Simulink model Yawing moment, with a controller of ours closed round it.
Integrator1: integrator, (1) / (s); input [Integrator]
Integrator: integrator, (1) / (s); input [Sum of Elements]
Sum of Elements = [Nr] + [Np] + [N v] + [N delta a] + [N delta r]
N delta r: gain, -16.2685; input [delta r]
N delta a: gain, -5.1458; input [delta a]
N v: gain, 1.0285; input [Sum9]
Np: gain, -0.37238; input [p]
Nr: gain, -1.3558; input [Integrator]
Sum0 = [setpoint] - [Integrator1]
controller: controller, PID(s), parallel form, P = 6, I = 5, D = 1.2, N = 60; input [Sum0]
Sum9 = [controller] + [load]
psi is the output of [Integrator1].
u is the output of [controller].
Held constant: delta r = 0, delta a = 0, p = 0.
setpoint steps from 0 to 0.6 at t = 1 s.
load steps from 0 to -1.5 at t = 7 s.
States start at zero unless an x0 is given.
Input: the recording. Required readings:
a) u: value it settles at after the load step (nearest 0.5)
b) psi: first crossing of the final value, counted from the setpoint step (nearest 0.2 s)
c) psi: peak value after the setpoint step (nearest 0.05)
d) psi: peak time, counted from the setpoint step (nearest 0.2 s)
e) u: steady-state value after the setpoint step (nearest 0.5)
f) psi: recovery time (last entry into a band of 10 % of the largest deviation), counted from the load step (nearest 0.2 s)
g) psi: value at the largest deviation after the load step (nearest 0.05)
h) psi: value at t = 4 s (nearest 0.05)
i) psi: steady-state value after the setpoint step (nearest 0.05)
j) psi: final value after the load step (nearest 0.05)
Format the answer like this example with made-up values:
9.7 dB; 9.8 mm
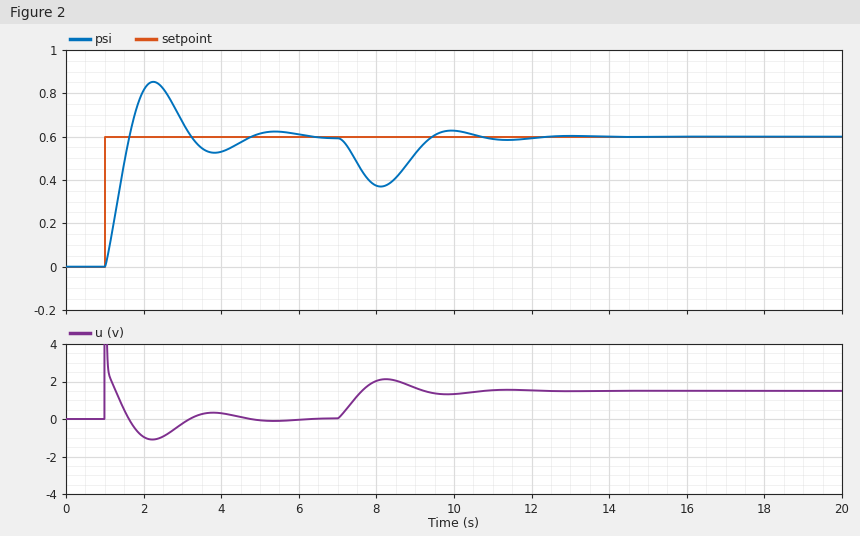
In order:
1.5; 0.6 s; 0.85; 1.2 s; 0.0; 3.2 s; 0.35; 0.55; 0.60; 0.60
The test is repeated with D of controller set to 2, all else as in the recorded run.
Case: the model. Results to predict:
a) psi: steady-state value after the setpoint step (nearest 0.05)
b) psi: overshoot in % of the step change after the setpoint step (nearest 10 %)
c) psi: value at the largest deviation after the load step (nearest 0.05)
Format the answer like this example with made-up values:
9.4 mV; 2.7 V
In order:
0.60; 30 %; 0.40
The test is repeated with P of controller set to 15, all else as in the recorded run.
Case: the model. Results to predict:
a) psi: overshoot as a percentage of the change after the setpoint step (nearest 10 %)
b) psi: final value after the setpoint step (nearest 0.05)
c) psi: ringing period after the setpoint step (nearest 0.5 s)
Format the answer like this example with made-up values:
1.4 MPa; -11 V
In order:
40 %; 0.60; 1.5 s
